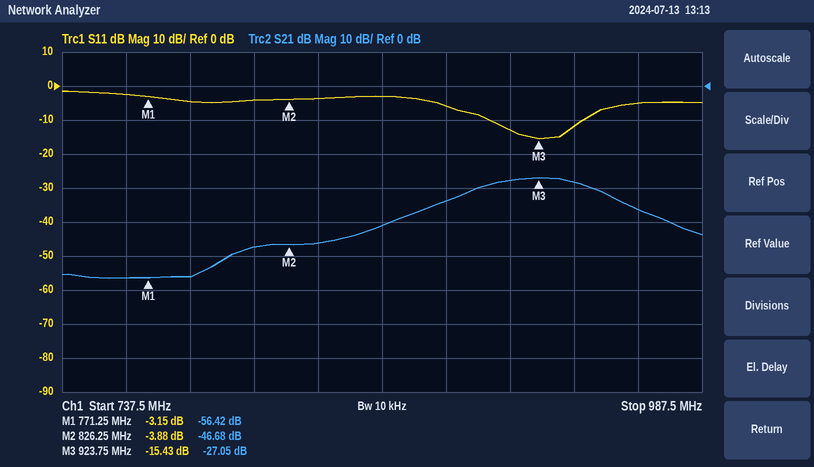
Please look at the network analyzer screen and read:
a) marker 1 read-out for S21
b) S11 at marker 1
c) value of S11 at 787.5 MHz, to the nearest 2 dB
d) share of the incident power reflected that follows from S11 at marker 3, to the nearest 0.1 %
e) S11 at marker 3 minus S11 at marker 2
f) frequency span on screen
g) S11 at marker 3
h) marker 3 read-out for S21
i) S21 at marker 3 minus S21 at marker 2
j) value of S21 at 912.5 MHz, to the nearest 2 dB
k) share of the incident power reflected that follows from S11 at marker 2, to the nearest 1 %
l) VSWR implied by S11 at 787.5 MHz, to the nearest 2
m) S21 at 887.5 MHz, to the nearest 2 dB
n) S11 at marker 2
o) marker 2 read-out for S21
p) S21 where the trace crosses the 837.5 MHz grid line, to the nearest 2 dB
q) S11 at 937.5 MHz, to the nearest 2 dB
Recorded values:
-56.42 dB
-3.15 dB
-4 dB
2.9 %
-11.55 dB
250 MHz
-15.43 dB
-27.05 dB
19.63 dB
-28 dB
41 %
4
-34 dB
-3.88 dB
-46.68 dB
-46 dB
-12 dB
